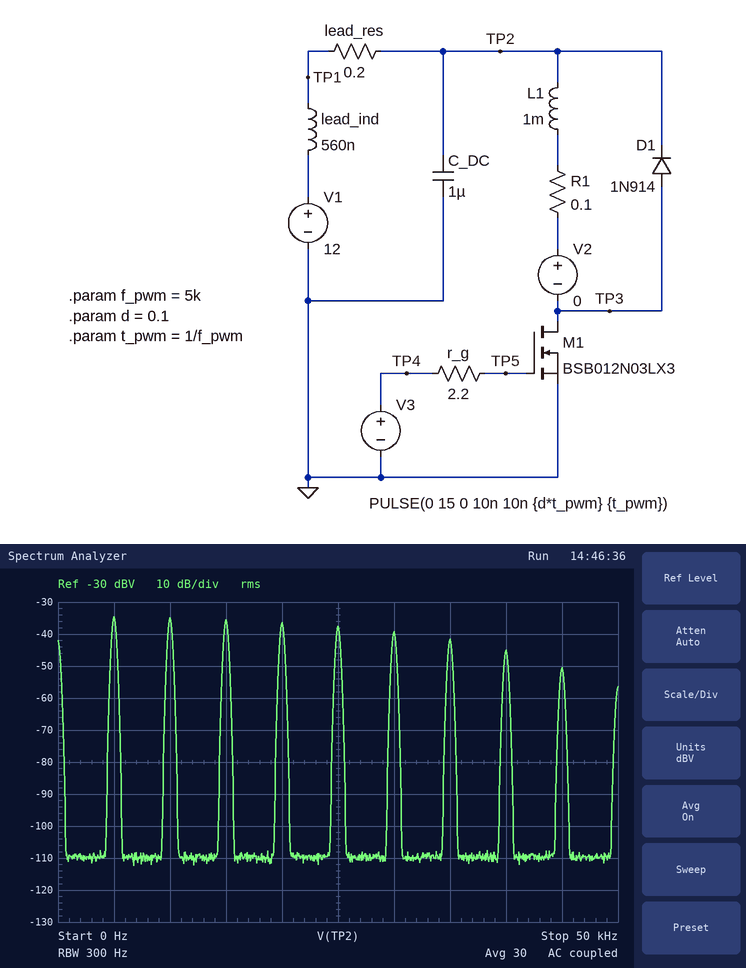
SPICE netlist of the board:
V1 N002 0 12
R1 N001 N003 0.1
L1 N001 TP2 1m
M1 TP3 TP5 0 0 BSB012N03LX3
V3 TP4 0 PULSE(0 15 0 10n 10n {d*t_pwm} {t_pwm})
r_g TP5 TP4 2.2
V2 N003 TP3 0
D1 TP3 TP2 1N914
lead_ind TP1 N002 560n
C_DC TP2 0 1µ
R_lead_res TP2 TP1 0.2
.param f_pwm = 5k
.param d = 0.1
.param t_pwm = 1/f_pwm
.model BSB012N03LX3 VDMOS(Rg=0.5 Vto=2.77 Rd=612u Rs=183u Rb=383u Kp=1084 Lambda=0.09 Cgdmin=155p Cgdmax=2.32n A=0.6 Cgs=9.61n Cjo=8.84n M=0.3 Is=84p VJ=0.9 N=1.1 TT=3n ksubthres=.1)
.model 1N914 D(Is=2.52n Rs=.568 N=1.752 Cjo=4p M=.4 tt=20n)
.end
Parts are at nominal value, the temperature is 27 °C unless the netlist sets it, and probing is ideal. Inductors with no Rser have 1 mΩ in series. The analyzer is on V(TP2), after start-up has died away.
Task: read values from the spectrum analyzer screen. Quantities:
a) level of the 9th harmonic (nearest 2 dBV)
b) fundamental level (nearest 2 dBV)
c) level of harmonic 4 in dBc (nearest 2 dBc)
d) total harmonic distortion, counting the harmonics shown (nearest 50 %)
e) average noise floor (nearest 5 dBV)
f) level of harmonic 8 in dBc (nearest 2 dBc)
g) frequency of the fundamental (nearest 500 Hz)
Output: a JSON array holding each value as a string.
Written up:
["-50 dBV", "-34 dBV", "-2 dBc", "200 %", "-110 dBV", "-10 dBc", "5.0 kHz"]
